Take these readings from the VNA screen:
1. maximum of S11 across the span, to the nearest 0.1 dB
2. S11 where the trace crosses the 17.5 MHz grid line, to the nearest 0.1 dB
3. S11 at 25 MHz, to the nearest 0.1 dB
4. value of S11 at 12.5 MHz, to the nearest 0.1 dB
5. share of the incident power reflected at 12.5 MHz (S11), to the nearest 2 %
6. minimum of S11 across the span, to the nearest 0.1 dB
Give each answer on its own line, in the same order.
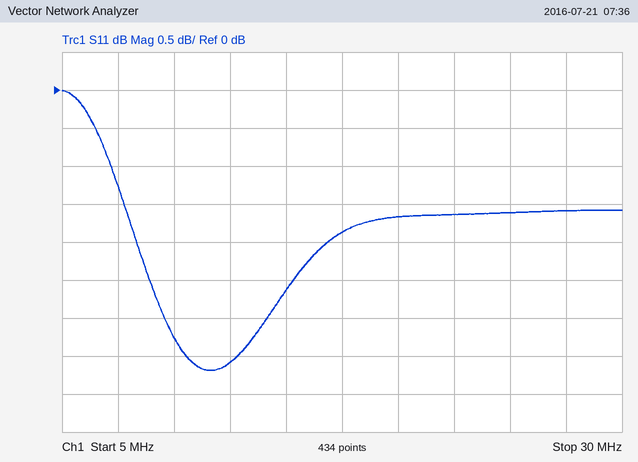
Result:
0.0 dB
-1.9 dB
-1.6 dB
-3.6 dB
44 %
-3.7 dB
